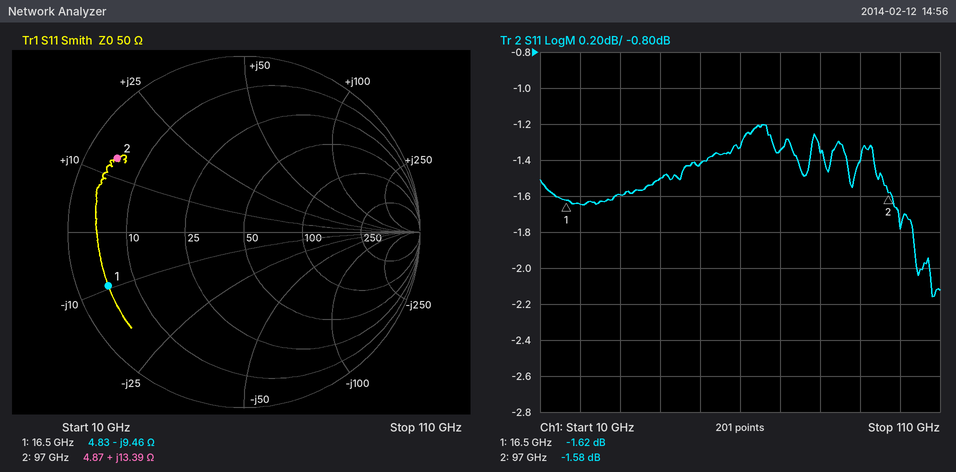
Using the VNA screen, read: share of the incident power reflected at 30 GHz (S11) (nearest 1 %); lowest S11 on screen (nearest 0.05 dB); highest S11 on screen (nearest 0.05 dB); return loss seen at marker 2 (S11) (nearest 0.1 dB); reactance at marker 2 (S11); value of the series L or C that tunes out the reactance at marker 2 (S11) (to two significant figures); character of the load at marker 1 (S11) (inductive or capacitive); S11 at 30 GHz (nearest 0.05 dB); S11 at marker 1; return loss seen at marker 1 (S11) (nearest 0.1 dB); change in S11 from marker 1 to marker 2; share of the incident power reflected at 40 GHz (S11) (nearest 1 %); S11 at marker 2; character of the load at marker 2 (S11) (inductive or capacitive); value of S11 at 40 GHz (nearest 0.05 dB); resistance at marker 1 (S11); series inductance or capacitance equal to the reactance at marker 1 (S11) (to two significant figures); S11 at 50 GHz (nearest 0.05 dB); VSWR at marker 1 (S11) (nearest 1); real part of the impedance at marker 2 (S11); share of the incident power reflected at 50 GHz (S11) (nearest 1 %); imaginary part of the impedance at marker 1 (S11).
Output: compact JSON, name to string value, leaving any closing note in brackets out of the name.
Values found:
{"share of the incident power reflected at 30 GHz (S11)": "69 %", "lowest S11 on screen": "-2.15 dB", "highest S11 on screen": "-1.20 dB", "return loss seen at marker 2 (S11)": "1.6 dB", "reactance at marker 2": "+13.39 Ω", "value of the series L or C that tunes out the reactance at marker 2 (S11)": "120 fF", "character of the load at marker 1 (S11)": "capacitive", "S11 at 30 GHz": "-1.60 dB", "S11 at marker 1": "-1.62 dB", "return loss seen at marker 1 (S11)": "1.6 dB", "change in S11 from marker 1 to marker 2": "0.04 dB", "share of the incident power reflected at 40 GHz (S11)": "71 %", "S11 at marker 2": "-1.58 dB", "character of the load at marker 2 (S11)": "inductive", "value of S11 at 40 GHz": "-1.50 dB", "resistance at marker 1": "4.83 Ω", "series inductance or capacitance equal to the reactance at marker 1 (S11)": "1.0 pF", "S11 at 50 GHz": "-1.40 dB", "VSWR at marker 1 (S11)": "11", "real part of the impedance at marker 2": "4.87 Ω", "share of the incident power reflected at 50 GHz (S11)": "72 %", "imaginary part of the impedance at marker 1": "-9.46 Ω"}
